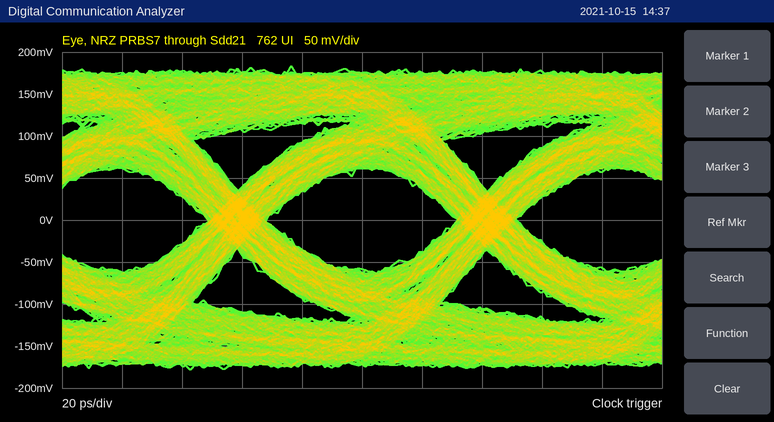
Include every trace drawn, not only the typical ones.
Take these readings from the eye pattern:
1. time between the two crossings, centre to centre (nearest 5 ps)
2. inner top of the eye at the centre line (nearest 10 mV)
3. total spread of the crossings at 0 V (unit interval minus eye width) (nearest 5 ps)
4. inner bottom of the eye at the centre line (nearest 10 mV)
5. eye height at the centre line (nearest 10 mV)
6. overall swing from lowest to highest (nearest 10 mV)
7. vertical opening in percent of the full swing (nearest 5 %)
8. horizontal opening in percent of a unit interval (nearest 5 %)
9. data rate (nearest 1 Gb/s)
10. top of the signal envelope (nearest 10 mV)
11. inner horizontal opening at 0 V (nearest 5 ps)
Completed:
85 ps
60 mV
20 ps
-60 mV
120 mV
360 mV
35 %
75 %
12 Gb/s
180 mV
65 ps
